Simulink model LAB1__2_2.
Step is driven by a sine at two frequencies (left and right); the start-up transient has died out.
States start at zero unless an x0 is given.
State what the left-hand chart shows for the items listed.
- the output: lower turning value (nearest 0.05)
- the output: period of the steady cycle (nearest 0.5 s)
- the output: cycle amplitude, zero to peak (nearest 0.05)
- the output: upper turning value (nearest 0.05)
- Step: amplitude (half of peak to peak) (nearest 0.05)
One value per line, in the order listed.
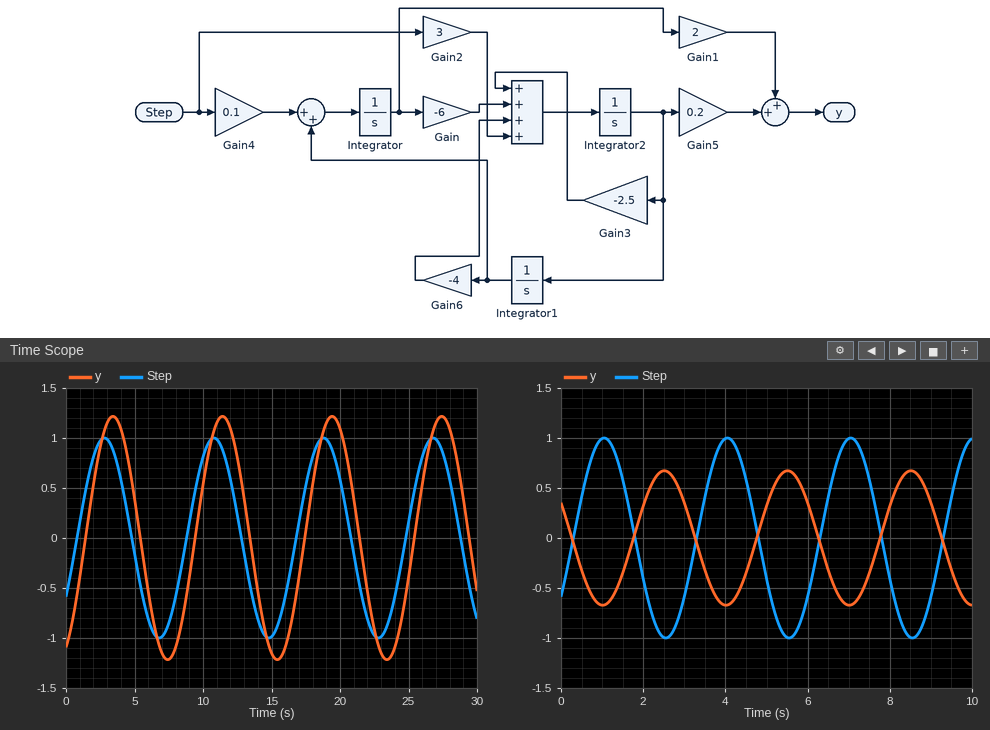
-1.20
8.0 s
1.20
1.20
1.00
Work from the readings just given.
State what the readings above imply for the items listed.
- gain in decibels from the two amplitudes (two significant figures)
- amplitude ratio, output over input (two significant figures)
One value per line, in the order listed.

1.6 dB
1.2
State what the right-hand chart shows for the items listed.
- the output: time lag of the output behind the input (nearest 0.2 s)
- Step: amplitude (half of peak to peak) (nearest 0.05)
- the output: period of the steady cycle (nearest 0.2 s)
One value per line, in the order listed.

1.4 s
1.00
3.0 s
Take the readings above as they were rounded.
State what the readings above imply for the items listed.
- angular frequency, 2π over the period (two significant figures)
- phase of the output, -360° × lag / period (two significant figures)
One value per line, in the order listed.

2.1 rad/s
-170°
